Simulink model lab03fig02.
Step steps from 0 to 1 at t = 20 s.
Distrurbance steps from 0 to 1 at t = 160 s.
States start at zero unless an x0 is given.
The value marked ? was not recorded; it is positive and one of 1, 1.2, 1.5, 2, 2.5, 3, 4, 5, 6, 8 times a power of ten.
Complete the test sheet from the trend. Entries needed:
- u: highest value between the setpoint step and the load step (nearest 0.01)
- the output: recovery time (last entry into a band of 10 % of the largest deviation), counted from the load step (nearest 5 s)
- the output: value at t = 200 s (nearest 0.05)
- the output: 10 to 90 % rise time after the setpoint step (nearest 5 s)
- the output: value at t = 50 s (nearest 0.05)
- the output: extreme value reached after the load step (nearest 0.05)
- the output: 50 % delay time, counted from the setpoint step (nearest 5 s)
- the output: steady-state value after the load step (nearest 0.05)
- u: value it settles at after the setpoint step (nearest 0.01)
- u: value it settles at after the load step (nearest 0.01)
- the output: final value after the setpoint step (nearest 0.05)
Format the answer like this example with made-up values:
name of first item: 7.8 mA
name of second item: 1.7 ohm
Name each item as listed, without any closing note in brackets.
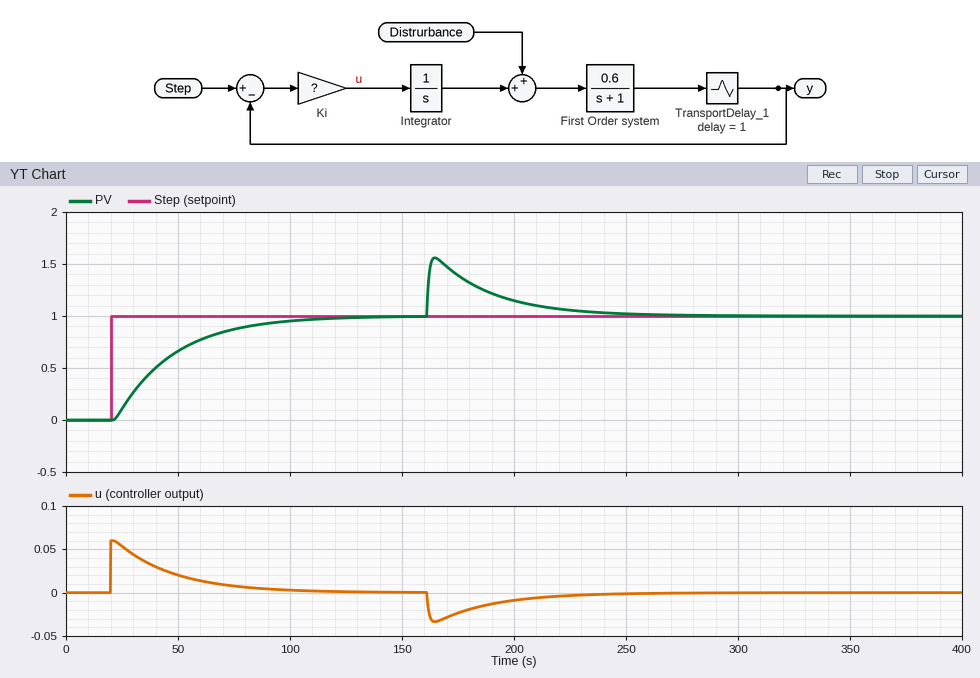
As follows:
u: highest value between the setpoint step and the load step: 0.06
the output: recovery time (last entry into a band of 10 % of the largest deviation), counted from the load step: 65 s
the output: value at t = 200 s: 1.15
the output: 10 to 90 % rise time after the setpoint step: 55 s
the output: value at t = 50 s: 0.65
the output: extreme value reached after the load step: 1.55
the output: 50 % delay time, counted from the setpoint step: 20 s
the output: steady-state value after the load step: 1.00
u: value it settles at after the setpoint step: 0.00
u: value it settles at after the load step: 0.00
the output: final value after the setpoint step: 1.00
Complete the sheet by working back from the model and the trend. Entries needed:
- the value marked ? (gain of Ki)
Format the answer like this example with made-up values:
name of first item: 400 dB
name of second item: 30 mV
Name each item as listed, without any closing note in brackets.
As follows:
the value marked ?: 0.06
